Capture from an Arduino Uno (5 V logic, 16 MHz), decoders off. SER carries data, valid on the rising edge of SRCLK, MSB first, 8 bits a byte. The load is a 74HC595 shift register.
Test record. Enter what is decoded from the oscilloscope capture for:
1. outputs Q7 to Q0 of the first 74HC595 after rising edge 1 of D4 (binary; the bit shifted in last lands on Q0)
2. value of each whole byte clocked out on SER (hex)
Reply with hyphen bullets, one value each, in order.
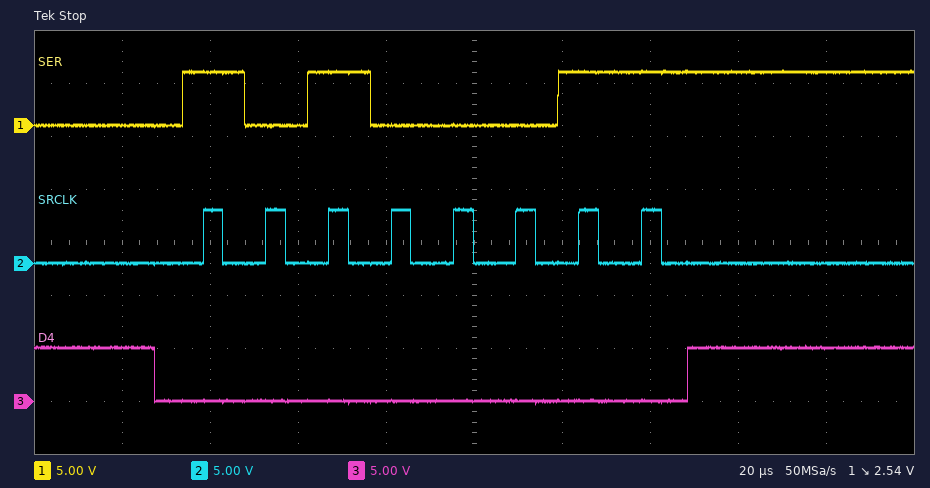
- 10100011
- 0xA3
